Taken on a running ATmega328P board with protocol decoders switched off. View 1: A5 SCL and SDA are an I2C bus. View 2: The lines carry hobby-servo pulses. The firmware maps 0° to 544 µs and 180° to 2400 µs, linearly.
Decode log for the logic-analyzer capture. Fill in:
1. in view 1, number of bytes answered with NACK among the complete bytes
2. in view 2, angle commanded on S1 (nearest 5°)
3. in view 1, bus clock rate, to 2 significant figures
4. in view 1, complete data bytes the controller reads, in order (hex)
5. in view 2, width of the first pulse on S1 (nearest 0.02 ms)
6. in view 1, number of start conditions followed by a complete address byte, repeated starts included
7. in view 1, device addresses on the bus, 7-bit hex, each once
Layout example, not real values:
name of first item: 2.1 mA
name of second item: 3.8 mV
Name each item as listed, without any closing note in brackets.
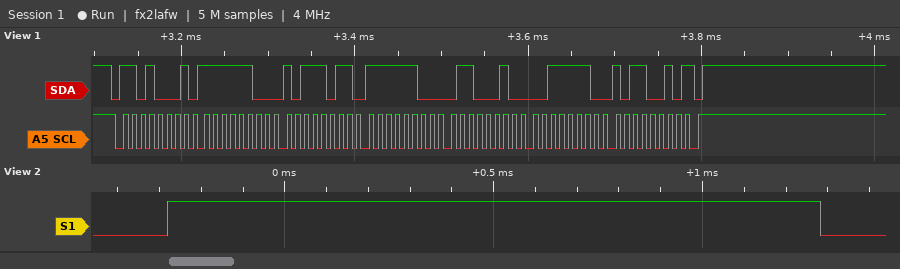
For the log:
in view 1, number of bytes answered with NACK among the complete bytes: 1
in view 2, angle commanded on S1: 100°
in view 1, bus clock rate, to 2 significant figures: 100 kHz
in view 1, complete data bytes the controller reads, in order: FC BB FC 62 3E B2
in view 2, width of the first pulse on S1: 1.56 ms
in view 1, number of start conditions followed by a complete address byte, repeated starts included: 1
in view 1, device addresses on the bus, 7-bit hex, each once: 0x68
